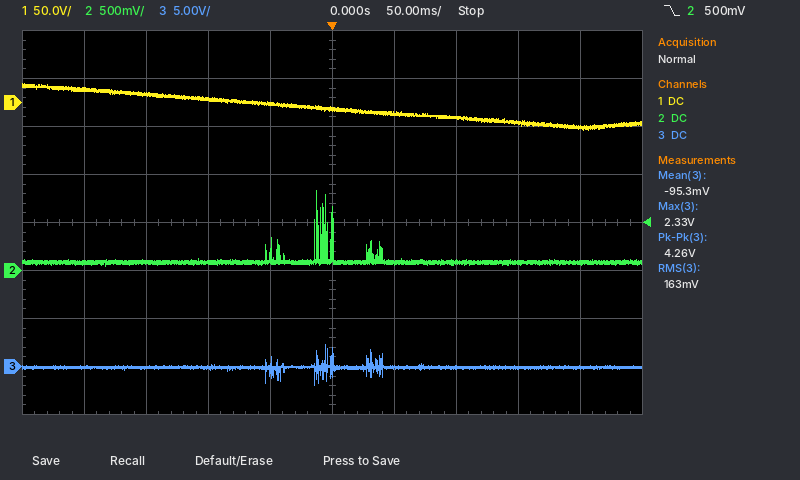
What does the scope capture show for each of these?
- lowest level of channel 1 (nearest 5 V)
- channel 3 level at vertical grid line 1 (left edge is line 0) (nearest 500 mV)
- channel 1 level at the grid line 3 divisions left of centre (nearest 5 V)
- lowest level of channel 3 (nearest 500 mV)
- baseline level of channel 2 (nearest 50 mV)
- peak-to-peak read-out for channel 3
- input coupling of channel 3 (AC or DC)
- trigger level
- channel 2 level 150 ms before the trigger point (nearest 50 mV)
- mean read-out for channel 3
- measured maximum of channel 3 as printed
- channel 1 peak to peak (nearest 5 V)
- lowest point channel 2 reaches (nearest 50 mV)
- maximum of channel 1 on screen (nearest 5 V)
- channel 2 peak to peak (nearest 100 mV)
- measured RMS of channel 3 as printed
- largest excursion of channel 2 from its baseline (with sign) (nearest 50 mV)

-30 V
0.0 V
10 V
-2.0 V
100 mV
4.26 V
DC
500 mV
100 mV
-95.3 mV
2.33 V
50 V
50 mV
20 V
800 mV
163 mV
+750 mV
